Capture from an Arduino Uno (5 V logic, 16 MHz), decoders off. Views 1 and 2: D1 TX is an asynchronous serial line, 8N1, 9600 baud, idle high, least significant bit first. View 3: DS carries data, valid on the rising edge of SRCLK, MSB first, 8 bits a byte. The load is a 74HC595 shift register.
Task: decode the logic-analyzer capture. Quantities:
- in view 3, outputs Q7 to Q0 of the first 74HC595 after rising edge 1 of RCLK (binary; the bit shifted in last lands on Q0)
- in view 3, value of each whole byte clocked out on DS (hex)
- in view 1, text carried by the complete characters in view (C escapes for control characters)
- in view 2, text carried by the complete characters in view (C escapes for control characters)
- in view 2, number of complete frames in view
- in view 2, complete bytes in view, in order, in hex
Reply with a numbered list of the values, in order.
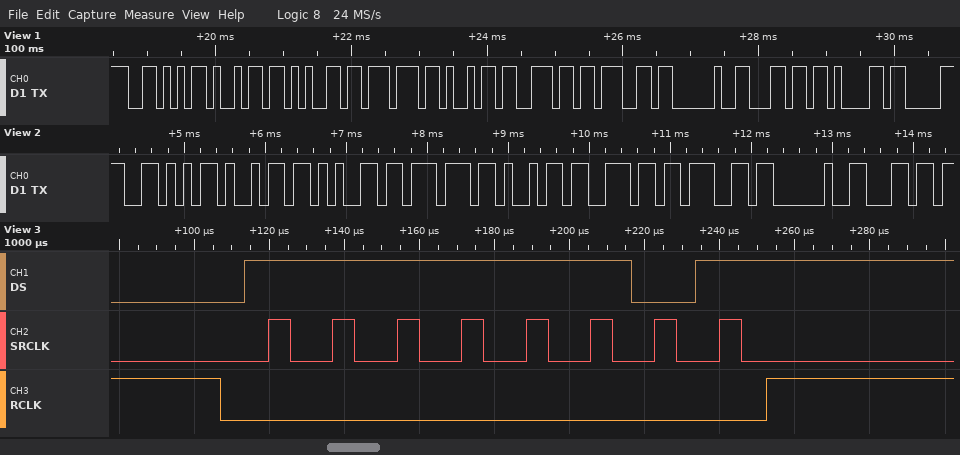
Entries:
1. 11111101
2. FD
3. "Viewing la"
4. "Viewing l"
5. 9
6. 56 69 65 77 69 6E 67 20 6C
